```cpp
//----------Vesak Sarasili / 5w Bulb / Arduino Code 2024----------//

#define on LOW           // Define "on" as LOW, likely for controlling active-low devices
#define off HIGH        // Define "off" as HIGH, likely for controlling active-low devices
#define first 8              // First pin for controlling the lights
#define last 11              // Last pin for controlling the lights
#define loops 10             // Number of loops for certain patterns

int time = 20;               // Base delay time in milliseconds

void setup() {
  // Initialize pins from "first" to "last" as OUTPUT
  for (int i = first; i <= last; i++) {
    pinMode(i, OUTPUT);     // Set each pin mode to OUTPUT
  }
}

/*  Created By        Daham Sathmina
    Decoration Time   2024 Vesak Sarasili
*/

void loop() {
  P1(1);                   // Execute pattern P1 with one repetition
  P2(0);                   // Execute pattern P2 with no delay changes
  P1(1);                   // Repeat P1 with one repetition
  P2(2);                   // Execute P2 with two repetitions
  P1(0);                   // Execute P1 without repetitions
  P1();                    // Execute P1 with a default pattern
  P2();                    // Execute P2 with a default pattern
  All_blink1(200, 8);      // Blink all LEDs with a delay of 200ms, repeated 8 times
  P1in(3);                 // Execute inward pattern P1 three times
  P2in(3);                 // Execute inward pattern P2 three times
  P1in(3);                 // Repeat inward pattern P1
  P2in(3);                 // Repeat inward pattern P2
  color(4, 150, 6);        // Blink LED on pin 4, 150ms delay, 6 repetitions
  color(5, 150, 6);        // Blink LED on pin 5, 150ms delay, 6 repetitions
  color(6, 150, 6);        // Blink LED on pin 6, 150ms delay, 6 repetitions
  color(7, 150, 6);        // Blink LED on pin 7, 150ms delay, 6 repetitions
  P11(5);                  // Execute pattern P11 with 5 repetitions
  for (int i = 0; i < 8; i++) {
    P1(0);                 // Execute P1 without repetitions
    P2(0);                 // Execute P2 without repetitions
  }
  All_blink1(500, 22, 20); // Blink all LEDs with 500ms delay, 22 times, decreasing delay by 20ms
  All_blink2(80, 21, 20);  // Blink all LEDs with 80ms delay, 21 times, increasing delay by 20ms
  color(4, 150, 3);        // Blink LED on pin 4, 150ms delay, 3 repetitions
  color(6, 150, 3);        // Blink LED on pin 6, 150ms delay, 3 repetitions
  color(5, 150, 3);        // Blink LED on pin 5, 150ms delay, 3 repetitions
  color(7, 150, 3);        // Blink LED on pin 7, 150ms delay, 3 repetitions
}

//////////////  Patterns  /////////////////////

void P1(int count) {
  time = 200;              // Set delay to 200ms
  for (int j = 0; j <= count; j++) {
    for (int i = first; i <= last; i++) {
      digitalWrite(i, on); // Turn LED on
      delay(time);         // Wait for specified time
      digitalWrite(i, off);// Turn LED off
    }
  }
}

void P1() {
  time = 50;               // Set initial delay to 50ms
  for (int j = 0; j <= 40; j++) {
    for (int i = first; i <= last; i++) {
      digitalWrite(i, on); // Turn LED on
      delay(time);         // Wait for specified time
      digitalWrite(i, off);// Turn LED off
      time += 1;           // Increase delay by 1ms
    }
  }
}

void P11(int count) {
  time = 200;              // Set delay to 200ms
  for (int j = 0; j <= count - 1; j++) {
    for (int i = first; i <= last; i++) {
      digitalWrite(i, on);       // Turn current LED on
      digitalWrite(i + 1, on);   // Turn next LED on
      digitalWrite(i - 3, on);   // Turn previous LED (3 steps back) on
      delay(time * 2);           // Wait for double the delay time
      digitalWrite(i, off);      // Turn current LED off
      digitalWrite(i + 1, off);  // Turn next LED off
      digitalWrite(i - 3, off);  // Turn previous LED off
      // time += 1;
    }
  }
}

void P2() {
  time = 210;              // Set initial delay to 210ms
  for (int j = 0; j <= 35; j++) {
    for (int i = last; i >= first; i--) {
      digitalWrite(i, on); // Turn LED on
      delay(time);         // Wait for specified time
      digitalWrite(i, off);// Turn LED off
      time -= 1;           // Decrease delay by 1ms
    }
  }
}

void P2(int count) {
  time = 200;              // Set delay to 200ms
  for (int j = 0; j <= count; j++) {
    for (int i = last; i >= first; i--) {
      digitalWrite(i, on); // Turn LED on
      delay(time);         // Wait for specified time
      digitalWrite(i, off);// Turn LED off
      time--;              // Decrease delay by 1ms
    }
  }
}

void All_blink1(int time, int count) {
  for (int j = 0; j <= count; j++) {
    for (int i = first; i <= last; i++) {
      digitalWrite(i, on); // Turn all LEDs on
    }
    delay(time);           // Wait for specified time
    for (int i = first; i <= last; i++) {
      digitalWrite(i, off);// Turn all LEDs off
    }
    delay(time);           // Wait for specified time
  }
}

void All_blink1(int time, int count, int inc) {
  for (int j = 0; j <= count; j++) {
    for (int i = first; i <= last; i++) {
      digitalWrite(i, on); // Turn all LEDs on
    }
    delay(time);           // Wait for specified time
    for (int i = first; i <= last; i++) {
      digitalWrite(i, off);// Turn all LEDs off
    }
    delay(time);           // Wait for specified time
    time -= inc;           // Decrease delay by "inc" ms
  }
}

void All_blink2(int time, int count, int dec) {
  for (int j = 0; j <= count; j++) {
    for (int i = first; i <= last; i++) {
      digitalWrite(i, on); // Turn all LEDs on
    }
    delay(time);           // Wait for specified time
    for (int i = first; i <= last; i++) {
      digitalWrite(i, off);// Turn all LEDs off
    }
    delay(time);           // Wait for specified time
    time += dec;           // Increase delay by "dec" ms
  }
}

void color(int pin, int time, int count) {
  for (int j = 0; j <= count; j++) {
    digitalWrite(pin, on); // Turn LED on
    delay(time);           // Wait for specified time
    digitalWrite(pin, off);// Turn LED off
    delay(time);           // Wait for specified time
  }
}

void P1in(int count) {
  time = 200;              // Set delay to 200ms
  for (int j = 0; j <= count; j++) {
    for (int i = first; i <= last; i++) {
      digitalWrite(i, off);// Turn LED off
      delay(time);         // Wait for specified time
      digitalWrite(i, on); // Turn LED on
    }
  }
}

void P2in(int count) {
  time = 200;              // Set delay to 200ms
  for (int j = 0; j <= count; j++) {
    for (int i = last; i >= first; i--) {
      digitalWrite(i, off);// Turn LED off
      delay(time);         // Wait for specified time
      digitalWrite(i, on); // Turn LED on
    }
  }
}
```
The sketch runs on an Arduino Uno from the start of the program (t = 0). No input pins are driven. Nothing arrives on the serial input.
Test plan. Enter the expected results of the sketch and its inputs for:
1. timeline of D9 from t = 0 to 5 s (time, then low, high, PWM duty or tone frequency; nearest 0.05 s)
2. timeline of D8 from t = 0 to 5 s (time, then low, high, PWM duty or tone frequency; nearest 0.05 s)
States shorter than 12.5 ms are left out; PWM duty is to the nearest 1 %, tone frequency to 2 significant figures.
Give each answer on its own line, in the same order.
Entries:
0 s low; 0.4 s high; 1 s low; 1.2 s high; 2 s low; 2.2 s high; 2.6 s low; 2.8 s high; 3.4 s low; 3.6 s high; 4.4 s low; 4.6 s high
0 s low; 0.2 s high; 0.8 s low; 1 s high; 2.2 s low; 2.6 s high; 3.2 s low; 3.4 s high; 4.6 s low; 4.8 s high
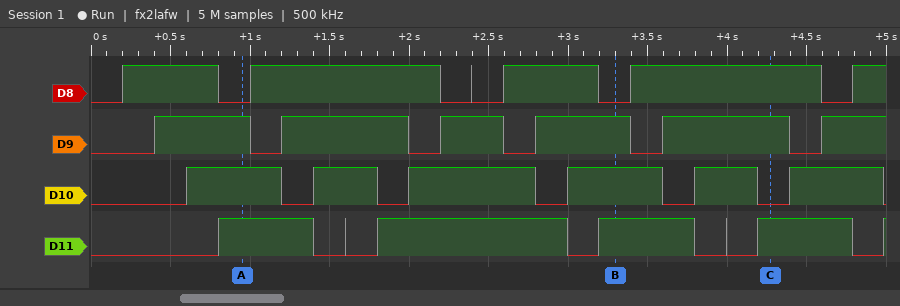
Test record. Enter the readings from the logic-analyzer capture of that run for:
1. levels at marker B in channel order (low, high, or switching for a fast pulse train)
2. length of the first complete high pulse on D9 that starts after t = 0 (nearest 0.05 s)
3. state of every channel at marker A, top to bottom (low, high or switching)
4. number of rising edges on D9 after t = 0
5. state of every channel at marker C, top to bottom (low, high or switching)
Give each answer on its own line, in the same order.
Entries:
D8 low, D9 high, D10 high, D11 high
0.60 s
D8 low, D9 high, D10 high, D11 high
6
D8 high, D9 high, D10 low, D11 high
